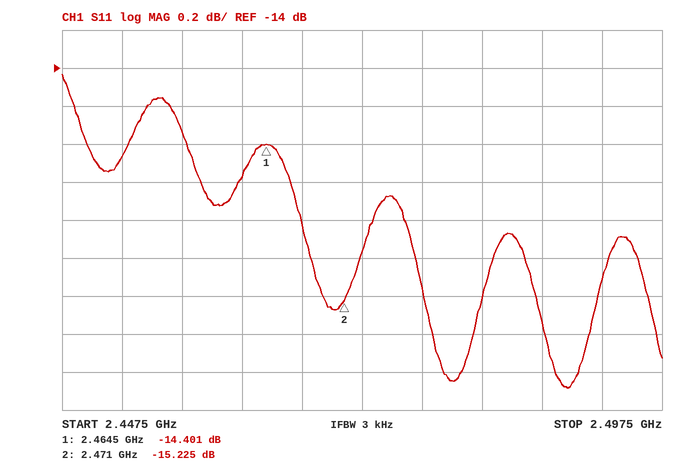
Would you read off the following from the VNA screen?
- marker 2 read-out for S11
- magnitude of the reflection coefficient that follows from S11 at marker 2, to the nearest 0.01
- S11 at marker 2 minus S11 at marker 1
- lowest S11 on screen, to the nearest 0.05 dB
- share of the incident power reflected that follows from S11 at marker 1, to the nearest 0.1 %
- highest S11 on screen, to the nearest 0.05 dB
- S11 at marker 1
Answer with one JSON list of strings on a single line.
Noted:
["-15.225 dB", "0.17", "-0.824 dB", "-15.70 dB", "3.6 %", "-14.05 dB", "-14.401 dB"]
